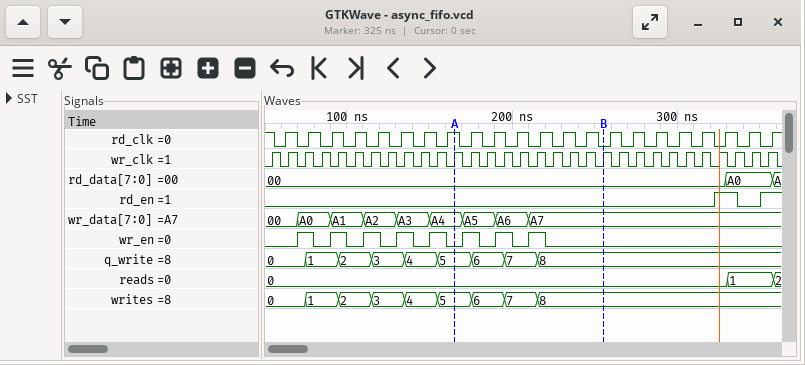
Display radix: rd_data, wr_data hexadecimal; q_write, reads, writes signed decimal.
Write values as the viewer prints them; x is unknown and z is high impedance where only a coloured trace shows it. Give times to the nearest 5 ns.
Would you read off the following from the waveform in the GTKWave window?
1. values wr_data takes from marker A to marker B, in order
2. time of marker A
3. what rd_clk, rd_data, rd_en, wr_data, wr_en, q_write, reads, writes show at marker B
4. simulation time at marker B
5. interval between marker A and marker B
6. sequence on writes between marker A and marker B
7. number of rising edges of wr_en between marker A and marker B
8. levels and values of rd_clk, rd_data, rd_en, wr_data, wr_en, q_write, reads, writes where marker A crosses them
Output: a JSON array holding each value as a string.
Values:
["A4, A5, A6, A7", "165 ns", "rd_clk=0, rd_data=00, rd_en=0, wr_data=A7, wr_en=0, q_write=8, reads=0, writes=8", "255 ns", "90 ns", "5, 6, 7, 8", "3", "rd_clk=1, rd_data=00, rd_en=0, wr_data=A4, wr_en=0, q_write=5, reads=0, writes=5"]
